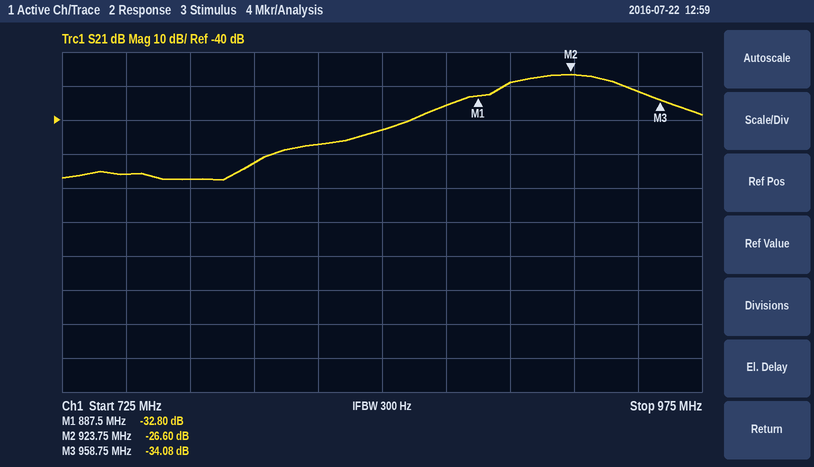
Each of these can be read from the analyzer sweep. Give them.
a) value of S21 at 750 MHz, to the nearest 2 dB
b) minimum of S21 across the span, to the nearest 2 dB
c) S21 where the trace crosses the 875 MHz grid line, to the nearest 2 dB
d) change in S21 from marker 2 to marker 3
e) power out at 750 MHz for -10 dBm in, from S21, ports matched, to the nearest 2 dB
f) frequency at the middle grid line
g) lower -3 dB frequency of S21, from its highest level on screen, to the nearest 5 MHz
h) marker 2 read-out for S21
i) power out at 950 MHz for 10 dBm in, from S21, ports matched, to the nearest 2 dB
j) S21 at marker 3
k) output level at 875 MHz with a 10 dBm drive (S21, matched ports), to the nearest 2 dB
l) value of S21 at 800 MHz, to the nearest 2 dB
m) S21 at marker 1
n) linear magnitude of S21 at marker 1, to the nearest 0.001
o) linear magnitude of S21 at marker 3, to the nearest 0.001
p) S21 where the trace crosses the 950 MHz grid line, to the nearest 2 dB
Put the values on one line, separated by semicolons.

-56 dB; -58 dB; -36 dB; -7.48 dB; -66 dBm; 850 MHz; 900 MHz; -26.60 dB; -22 dBm; -34.08 dB; -26 dBm; -52 dB; -32.80 dB; 0.023; 0.020; -32 dB
